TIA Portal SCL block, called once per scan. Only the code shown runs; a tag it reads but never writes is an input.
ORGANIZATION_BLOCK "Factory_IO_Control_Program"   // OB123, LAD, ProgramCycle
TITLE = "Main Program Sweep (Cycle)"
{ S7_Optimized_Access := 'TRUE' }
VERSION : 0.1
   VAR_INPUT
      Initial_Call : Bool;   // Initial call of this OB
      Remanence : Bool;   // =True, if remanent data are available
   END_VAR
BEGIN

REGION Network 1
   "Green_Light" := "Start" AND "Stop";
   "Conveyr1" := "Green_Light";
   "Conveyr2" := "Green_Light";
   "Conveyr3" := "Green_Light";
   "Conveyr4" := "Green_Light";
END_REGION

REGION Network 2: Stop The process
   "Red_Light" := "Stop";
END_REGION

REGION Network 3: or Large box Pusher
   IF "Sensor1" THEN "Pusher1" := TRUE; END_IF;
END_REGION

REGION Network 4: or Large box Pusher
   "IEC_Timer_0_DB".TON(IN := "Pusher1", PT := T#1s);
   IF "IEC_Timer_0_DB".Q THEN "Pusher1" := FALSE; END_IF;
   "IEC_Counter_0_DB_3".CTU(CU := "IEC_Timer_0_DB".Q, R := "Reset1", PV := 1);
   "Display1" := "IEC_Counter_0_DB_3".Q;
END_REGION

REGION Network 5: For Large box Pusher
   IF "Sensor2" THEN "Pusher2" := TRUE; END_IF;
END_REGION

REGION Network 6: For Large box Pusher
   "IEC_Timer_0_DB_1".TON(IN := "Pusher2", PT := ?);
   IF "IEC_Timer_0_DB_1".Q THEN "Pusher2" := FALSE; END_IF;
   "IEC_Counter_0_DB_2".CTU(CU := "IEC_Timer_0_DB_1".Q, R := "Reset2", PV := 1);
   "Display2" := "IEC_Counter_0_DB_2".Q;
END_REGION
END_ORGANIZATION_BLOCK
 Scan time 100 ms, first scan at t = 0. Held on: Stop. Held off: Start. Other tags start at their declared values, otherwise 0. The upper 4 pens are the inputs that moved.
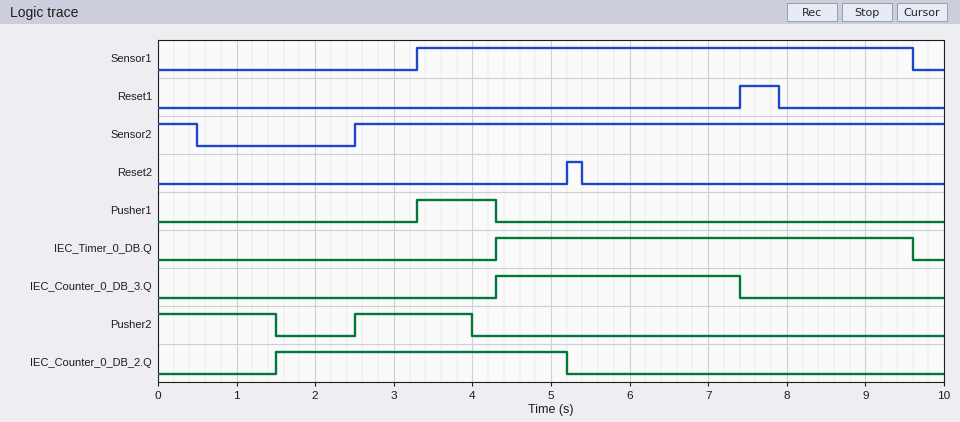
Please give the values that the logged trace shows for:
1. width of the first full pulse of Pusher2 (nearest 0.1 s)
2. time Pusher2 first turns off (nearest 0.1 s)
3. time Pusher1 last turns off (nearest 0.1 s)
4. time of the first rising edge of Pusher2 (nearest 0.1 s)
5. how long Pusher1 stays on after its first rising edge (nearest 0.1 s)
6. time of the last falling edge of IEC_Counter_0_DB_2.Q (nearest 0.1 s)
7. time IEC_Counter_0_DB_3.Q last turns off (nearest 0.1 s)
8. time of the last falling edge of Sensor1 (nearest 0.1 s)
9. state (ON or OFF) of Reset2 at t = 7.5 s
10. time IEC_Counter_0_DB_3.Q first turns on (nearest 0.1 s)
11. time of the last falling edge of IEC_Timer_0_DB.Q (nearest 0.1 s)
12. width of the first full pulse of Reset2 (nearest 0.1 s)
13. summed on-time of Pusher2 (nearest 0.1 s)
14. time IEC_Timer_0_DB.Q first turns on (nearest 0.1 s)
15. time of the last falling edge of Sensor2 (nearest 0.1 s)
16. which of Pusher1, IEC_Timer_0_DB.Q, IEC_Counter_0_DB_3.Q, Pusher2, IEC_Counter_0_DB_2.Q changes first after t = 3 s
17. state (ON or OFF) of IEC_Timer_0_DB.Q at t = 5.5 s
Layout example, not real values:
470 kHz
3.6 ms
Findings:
1.5 s
1.5 s
4.3 s
2.5 s
1.0 s
5.2 s
7.4 s
9.6 s
OFF
4.3 s
9.6 s
0.2 s
3.0 s
4.3 s
0.5 s
Pusher1
ON
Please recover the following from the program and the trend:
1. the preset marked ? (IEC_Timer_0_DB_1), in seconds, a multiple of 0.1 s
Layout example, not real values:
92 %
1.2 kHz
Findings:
1.5 s
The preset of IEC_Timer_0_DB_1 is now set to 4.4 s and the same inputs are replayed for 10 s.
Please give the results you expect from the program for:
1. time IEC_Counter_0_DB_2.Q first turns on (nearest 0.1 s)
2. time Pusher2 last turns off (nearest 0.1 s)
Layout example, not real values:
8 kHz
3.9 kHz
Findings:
4.4 s
4.4 s
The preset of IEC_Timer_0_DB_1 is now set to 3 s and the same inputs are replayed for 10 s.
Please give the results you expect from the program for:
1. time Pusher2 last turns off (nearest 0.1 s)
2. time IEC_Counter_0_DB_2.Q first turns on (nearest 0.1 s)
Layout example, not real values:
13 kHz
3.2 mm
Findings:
3.0 s
3.0 s
